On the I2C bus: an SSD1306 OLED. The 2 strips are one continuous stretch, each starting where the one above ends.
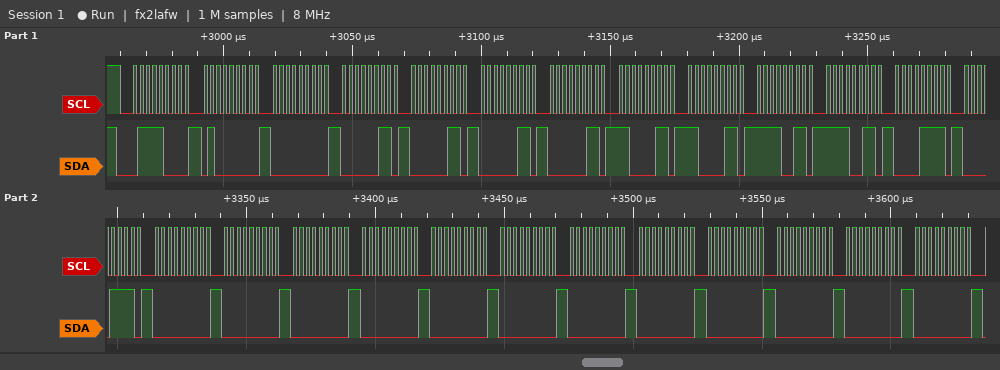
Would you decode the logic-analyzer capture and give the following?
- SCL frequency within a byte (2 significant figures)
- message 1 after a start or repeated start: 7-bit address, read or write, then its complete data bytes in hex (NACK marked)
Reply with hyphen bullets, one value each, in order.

- 400 kHz
- 0x3C write: 40 00 03 03 03 03 C3 C3 F3 F3 0F 0F 00 00 00 00 00 00 00 00 00 00 00 00
